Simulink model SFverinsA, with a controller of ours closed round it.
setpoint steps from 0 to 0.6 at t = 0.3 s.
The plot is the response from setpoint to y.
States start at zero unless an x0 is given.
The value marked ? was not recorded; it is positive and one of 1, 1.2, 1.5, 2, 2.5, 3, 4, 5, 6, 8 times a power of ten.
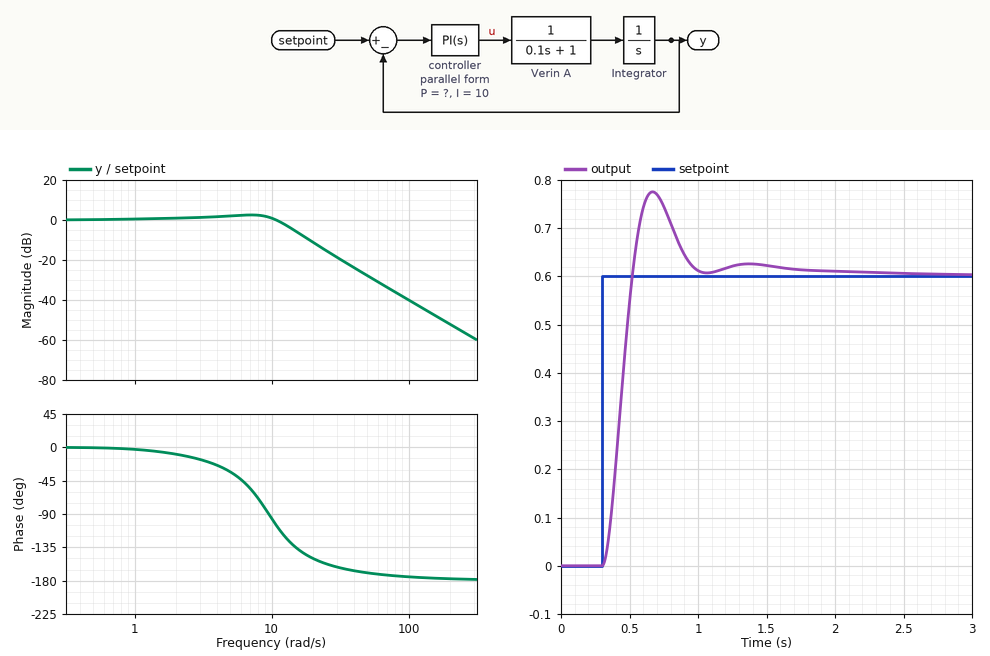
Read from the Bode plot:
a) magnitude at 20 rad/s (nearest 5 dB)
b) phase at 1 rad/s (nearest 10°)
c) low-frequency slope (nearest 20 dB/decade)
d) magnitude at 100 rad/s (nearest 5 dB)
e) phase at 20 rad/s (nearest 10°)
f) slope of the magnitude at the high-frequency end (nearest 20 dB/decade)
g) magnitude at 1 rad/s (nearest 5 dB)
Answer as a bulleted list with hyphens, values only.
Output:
- -10 dB
- 0°
- 0 dB/decade
- -40 dB
- -150°
- -40 dB/decade
- 0 dB
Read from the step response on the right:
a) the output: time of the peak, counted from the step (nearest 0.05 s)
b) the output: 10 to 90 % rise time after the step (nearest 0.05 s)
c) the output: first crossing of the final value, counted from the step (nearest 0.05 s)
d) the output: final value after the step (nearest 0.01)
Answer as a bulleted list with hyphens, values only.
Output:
- 0.35 s
- 0.15 s
- 0.20 s
- 0.60
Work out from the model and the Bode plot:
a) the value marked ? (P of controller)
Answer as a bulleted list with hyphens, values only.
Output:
- 10
